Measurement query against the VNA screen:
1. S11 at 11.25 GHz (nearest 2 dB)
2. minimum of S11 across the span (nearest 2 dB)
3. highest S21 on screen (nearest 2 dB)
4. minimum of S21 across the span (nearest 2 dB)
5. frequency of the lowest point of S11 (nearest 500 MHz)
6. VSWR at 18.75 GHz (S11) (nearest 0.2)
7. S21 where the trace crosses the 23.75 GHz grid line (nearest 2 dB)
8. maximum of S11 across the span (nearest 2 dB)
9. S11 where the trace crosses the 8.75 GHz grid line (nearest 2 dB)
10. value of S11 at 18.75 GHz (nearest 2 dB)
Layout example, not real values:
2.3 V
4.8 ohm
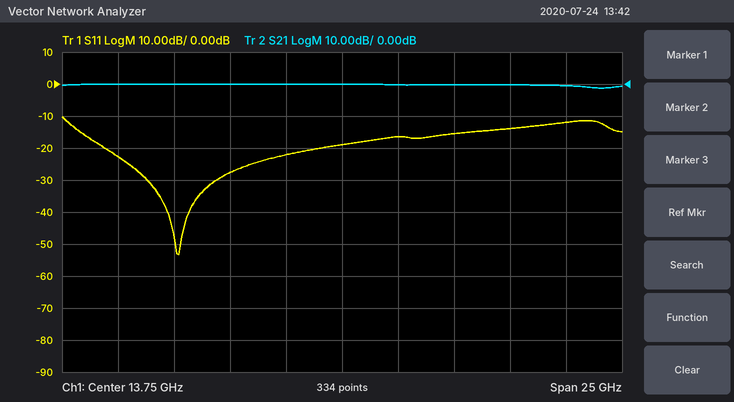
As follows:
-22 dB
-54 dB
0 dB
-2 dB
6.5 GHz
1.4
0 dB
-10 dB
-28 dB
-16 dB
